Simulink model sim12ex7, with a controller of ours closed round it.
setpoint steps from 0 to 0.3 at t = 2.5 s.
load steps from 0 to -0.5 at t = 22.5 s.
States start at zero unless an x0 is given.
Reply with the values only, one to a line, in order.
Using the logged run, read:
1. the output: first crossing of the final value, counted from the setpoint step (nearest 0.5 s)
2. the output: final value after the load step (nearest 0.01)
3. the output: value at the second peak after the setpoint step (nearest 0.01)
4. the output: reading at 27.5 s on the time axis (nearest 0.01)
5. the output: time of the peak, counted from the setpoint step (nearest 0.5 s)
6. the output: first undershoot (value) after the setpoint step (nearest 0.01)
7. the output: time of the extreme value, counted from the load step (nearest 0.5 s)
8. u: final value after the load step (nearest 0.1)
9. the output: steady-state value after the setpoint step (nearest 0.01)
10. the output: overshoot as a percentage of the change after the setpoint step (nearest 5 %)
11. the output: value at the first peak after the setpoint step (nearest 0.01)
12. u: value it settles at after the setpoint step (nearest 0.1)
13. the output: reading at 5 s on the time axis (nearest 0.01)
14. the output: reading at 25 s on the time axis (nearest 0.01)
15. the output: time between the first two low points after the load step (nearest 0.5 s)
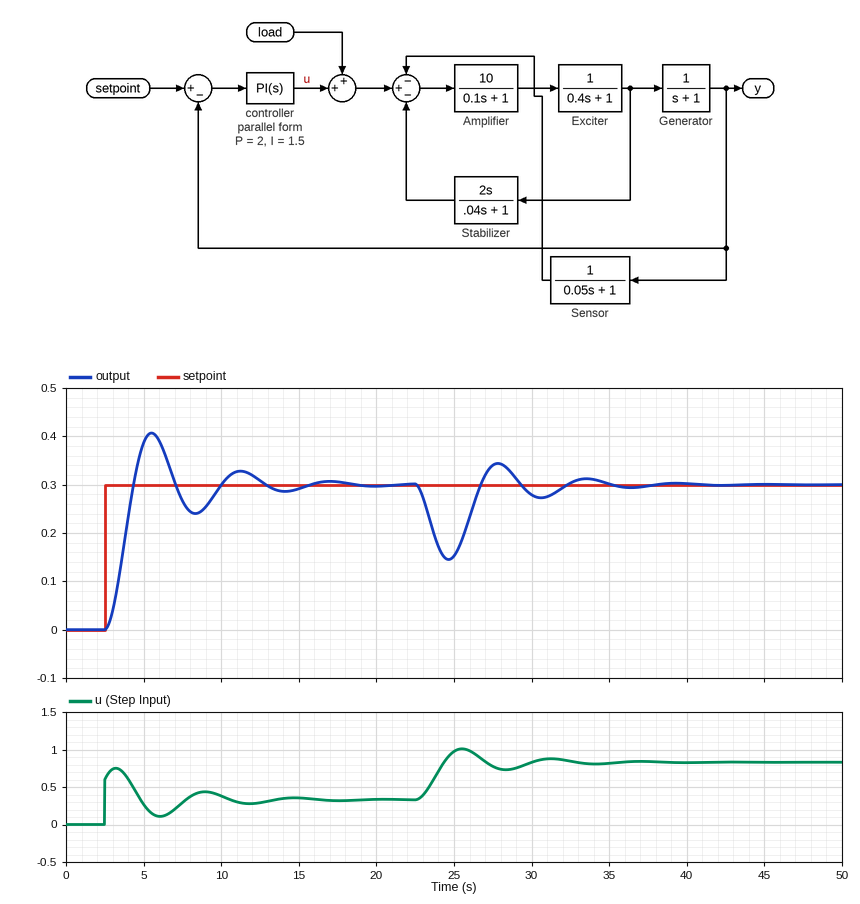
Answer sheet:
2.0 s
0.30
0.33
0.34
3.0 s
0.24
2.0 s
0.8
0.30
35 %
0.41
0.3
0.39
0.15
6.0 s
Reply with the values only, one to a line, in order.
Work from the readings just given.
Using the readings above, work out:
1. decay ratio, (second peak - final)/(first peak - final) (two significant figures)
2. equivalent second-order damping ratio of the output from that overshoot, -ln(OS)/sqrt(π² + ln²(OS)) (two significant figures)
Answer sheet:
0.27
0.32
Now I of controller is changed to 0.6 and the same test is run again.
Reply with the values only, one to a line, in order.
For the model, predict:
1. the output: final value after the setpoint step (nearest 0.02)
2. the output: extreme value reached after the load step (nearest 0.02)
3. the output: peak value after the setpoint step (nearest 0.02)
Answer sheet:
0.30
0.12
0.32
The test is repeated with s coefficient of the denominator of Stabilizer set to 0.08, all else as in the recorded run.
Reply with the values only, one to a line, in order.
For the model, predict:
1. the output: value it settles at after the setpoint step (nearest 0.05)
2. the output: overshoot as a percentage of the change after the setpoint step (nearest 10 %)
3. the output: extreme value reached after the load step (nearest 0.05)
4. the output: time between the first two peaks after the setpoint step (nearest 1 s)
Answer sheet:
0.30
30 %
0.15
6 s
